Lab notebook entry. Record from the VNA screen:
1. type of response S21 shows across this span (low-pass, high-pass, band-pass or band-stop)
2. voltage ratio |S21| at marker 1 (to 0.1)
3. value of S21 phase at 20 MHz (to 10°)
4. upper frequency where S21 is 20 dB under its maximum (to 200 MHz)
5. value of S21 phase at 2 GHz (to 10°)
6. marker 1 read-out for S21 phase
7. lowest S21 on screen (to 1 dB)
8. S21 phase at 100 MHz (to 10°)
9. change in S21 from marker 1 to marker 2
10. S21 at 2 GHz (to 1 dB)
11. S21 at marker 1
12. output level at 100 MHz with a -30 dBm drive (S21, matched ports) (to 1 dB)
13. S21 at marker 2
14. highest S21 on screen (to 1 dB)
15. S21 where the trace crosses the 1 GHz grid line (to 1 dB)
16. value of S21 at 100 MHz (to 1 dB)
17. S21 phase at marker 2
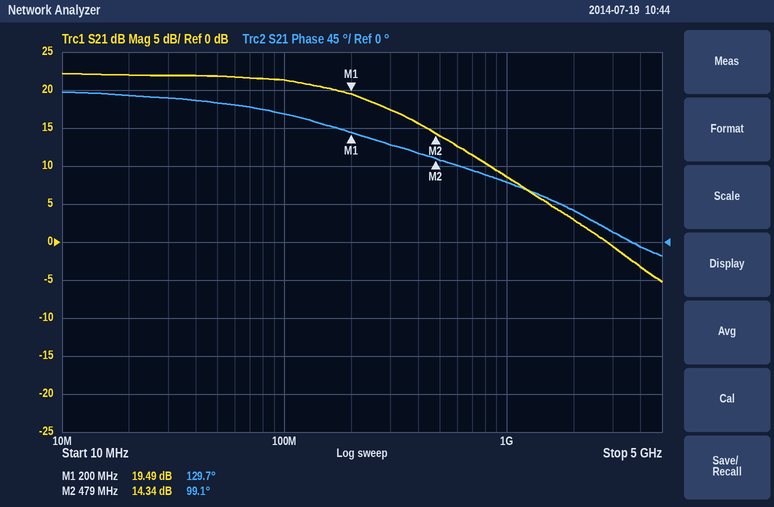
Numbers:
low-pass
9.4
170°
2.2 GHz
40°
129.7°
-5 dB
150°
-5.15 dB
3 dB
19.49 dB
-9 dBm
14.34 dB
22 dB
9 dB
21 dB
99.1°
